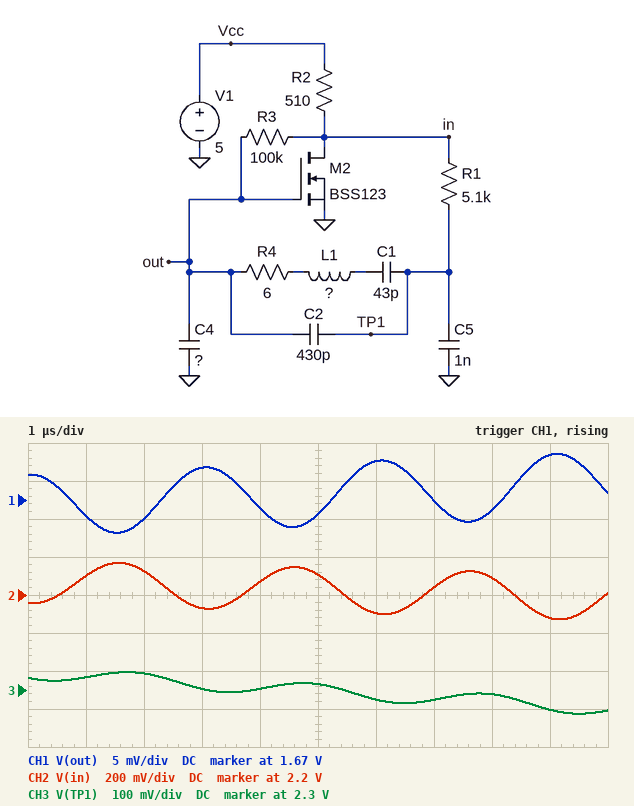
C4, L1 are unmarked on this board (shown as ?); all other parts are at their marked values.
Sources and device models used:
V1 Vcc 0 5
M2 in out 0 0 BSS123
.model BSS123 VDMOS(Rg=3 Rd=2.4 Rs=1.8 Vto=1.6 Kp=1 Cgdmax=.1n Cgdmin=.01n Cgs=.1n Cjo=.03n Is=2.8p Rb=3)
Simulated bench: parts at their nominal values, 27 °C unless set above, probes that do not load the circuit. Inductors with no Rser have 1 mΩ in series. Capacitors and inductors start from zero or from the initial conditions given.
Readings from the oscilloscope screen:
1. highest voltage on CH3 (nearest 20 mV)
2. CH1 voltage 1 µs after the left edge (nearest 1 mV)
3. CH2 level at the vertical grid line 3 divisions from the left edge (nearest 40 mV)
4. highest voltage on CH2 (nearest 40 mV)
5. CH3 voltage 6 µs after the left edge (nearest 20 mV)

2.34 V
1.668 V
2.12 V
2.36 V
2.28 V
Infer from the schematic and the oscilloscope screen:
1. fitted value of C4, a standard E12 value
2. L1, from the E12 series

2.2 nF
5.6 mH
